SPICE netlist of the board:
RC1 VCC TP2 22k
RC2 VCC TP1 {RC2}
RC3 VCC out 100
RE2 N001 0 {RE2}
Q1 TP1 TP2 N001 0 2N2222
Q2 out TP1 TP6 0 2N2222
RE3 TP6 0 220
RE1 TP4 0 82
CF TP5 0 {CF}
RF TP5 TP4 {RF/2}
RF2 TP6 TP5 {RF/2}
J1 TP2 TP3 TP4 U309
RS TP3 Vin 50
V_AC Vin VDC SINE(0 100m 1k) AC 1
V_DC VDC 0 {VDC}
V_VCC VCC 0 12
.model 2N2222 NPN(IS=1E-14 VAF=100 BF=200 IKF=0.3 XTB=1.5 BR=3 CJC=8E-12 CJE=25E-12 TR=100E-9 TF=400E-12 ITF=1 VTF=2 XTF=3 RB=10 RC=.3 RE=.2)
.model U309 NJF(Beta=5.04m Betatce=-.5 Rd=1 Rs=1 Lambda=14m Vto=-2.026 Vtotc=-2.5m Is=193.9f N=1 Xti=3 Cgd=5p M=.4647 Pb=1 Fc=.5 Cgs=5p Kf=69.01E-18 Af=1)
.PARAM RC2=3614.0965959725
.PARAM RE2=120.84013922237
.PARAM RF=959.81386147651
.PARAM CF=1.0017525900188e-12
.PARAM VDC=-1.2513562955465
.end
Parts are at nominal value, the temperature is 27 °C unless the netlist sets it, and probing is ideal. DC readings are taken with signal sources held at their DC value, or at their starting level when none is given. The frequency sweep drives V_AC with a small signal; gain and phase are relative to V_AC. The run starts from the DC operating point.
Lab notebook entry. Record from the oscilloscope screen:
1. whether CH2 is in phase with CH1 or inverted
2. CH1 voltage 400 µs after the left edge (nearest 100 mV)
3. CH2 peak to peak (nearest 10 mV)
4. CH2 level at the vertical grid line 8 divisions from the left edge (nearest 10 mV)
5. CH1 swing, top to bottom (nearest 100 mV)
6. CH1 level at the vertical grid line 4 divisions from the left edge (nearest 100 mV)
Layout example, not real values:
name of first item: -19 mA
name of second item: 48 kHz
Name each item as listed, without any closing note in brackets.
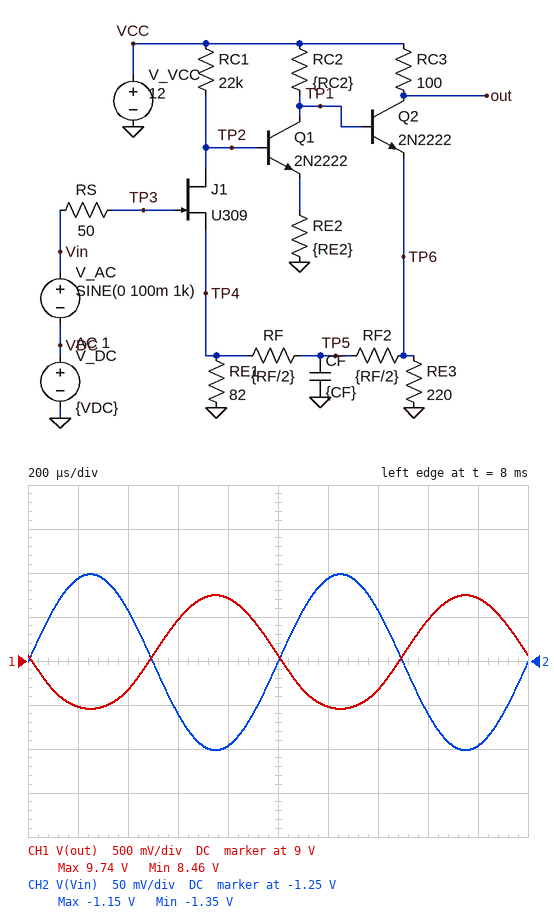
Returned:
whether CH2 is in phase with CH1 or inverted: inverted
CH1 voltage 400 µs after the left edge: 8.7 V
CH2 peak to peak: 200 mV
CH2 level at the vertical grid line 8 divisions from the left edge: -1.31 V
CH1 swing, top to bottom: 1.3 V
CH1 level at the vertical grid line 4 divisions from the left edge: 9.7 V
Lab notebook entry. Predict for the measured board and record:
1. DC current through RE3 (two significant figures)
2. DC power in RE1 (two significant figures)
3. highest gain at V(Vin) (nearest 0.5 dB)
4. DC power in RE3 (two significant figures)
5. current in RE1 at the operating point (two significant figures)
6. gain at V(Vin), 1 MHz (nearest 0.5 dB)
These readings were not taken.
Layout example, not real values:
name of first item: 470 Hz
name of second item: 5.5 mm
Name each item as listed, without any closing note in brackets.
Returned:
DC current through RE3: 24 mA
DC power in RE1: 2.6 mW
highest gain at V(Vin): 0 dB
DC power in RE3: 130 mW
current in RE1 at the operating point: 5.6 mA
gain at V(Vin), 1 MHz: 0 dB
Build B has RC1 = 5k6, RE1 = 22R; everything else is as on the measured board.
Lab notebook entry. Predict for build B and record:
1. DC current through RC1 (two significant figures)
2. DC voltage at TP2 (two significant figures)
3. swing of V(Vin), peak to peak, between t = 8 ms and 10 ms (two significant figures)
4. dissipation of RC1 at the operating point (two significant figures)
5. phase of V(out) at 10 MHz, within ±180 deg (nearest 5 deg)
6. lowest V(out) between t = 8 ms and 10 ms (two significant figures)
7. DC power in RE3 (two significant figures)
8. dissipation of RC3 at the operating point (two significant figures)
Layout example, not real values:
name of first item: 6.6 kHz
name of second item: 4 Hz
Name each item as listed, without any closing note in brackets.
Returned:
DC current through RC1: 2.0 mA
DC voltage at TP2: 870 mV
swing of V(Vin), peak to peak, between t = 8 ms and 10 ms: 200 mV
dissipation of RC1 at the operating point: 22 mW
phase of V(out) at 10 MHz, within ±180 deg: 85 deg
lowest V(out) between t = 8 ms and 10 ms: 7.8 V
DC power in RE3: 100 mW
dissipation of RC3 at the operating point: 69 mW
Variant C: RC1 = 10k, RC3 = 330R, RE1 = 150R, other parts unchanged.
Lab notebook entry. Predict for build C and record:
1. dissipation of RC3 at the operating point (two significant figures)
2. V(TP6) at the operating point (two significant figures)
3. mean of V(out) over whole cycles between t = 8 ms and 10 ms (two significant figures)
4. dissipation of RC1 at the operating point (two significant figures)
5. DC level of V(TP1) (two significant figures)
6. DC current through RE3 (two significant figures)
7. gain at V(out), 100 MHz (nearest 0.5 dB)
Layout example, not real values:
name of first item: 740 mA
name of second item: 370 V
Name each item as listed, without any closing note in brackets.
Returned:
dissipation of RC3 at the operating point: 15 mW
V(TP6) at the operating point: 1.3 V
mean of V(out) over whole cycles between t = 8 ms and 10 ms: 9.8 V
dissipation of RC1 at the operating point: 12 mW
DC level of V(TP1): 2.0 V
DC current through RE3: 5.8 mA
gain at V(out), 100 MHz: -4.5 dB
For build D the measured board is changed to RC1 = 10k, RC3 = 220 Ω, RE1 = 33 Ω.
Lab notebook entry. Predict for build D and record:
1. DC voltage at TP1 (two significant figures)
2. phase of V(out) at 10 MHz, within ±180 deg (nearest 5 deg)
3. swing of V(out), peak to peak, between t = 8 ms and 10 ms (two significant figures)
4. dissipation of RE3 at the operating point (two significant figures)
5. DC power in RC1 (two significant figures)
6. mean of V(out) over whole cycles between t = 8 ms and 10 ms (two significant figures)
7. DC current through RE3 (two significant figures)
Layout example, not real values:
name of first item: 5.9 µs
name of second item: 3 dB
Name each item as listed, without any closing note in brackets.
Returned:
DC voltage at TP1: 6.3 V
phase of V(out) at 10 MHz, within ±180 deg: -110 deg
swing of V(out), peak to peak, between t = 8 ms and 10 ms: 230 mV
dissipation of RE3 at the operating point: 140 mW
DC power in RC1: 13 mW
mean of V(out) over whole cycles between t = 8 ms and 10 ms: 5.6 V
DC current through RE3: 25 mA
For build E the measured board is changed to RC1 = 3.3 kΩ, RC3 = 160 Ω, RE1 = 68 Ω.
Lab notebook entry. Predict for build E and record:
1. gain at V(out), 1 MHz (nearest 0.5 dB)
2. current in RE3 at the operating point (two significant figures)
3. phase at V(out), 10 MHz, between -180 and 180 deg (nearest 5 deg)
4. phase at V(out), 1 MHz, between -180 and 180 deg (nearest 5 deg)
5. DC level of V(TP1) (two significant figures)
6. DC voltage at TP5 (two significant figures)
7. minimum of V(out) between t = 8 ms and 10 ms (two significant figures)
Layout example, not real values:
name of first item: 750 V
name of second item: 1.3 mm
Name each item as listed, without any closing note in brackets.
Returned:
gain at V(out), 1 MHz: -33.0 dB
current in RE3 at the operating point: 120 µA
phase at V(out), 10 MHz, between -180 and 180 deg: -70 deg
phase at V(out), 1 MHz, between -180 and 180 deg: -5 deg
DC level of V(TP1): 550 mV
DC voltage at TP5: 80 mV
minimum of V(out) between t = 8 ms and 10 ms: 12 V
